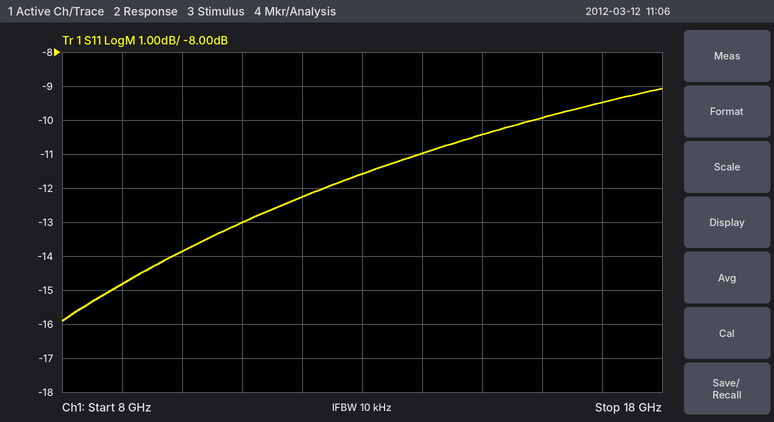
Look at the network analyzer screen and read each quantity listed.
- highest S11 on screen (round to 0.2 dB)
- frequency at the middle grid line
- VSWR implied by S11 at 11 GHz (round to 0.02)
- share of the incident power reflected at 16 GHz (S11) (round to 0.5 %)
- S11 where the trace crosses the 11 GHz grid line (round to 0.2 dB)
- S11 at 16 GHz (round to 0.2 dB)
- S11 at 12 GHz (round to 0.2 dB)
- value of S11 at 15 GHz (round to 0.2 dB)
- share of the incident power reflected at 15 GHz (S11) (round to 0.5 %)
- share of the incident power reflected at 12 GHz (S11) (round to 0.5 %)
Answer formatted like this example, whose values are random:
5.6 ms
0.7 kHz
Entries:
-9.0 dB
13 GHz
1.58
10.0 %
-13.0 dB
-10.0 dB
-12.2 dB
-10.4 dB
9.0 %
6.0 %
